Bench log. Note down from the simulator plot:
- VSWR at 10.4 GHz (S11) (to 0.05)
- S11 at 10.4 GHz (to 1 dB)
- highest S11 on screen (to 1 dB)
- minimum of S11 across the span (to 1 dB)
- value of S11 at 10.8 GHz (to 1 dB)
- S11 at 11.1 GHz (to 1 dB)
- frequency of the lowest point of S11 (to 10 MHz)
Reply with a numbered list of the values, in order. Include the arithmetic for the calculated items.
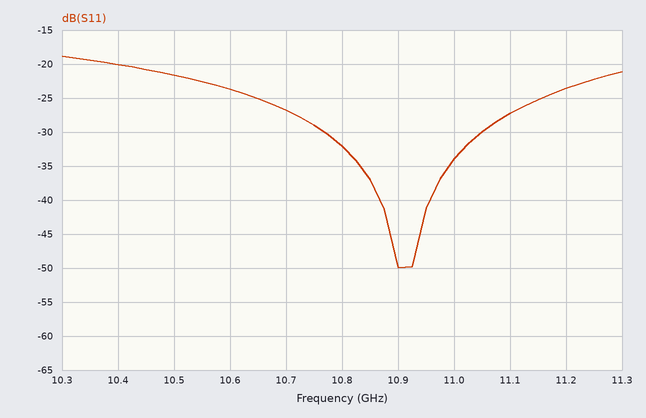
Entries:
1. |Γ| = 10^(-20/20) = 0.1000; VSWR = (1 + 0.1000)/(1 − 0.1000) ≈ 1.22, so 1.20 to the nearest 0.05
2. -20 dB
3. -19 dB
4. -50 dB
5. -32 dB
6. -27 dB
7. 10.90 GHz
